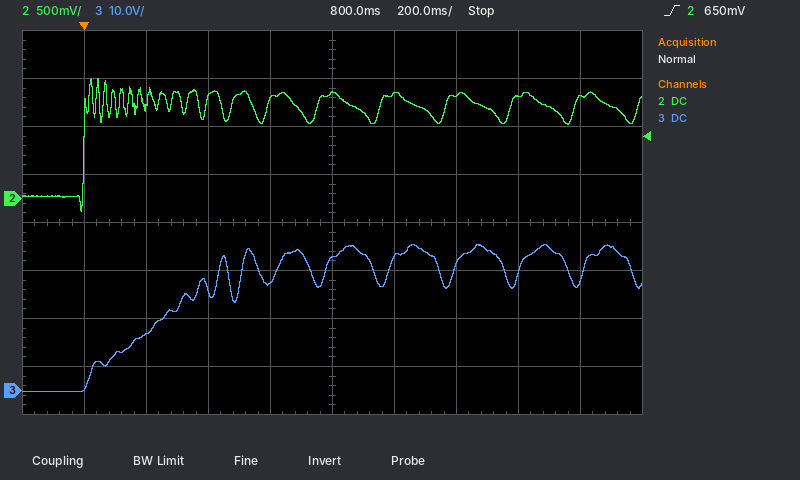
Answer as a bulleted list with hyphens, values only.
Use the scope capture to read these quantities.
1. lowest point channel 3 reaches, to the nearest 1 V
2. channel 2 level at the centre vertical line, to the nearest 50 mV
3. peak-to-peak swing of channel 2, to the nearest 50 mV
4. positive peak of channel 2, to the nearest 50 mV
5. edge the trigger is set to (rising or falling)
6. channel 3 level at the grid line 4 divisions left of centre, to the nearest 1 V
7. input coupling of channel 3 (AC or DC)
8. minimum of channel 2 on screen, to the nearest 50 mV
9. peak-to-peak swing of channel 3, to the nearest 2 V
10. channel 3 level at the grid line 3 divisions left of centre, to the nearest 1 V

- 0 V
- 1.10 V
- 1.40 V
- 1.25 V
- rising
- 1 V
- DC
- -150 mV
- 30 V
- 12 V
